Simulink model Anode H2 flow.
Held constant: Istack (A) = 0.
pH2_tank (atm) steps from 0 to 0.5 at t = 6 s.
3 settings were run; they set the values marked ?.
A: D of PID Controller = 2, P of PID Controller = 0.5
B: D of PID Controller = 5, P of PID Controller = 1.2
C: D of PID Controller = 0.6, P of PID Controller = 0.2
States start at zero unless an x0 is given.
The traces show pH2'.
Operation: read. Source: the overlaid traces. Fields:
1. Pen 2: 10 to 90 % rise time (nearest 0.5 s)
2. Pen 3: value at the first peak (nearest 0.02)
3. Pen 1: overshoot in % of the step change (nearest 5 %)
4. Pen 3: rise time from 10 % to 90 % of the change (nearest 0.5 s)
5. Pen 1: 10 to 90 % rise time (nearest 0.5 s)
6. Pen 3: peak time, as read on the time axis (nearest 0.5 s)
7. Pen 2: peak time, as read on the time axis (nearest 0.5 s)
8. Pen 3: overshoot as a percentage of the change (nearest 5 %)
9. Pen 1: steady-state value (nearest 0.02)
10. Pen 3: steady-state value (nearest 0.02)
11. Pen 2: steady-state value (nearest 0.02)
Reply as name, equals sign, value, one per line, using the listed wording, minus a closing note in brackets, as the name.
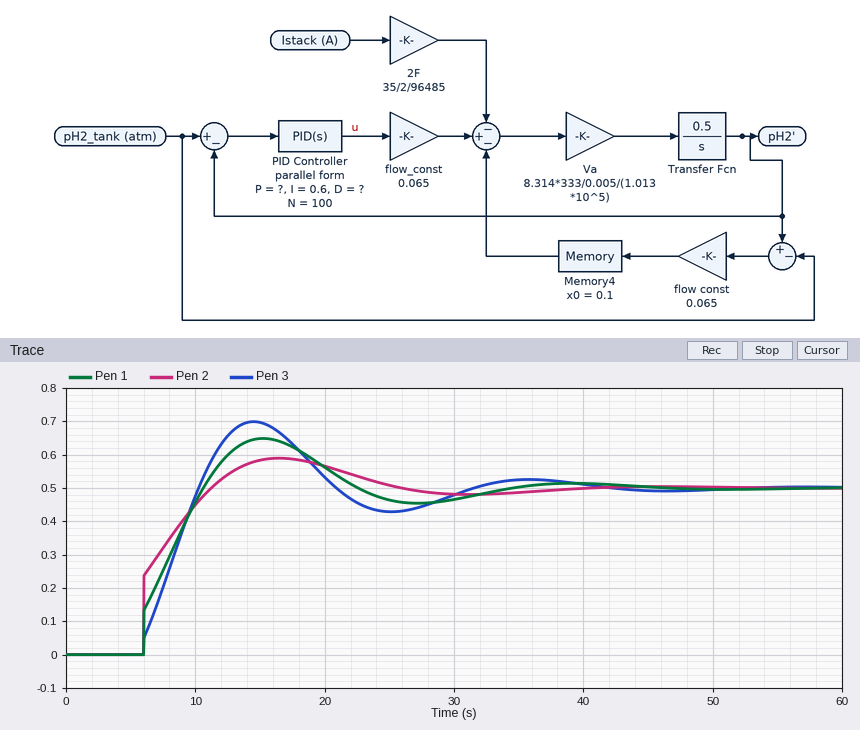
Pen 2: 10 to 90 % rise time = 4.0 s
Pen 3: value at the first peak = 0.70
Pen 1: overshoot in % of the step change = 30 %
Pen 3: rise time from 10 % to 90 % of the change = 3.5 s
Pen 1: 10 to 90 % rise time = 4.0 s
Pen 3: peak time, as read on the time axis = 14.5 s
Pen 2: peak time, as read on the time axis = 16.5 s
Pen 3: overshoot as a percentage of the change = 40 %
Pen 1: steady-state value = 0.50
Pen 3: steady-state value = 0.50
Pen 2: steady-state value = 0.50
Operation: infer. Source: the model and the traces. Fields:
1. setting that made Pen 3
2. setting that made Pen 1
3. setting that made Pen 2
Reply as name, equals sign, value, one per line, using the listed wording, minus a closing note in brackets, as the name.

setting that made Pen 3 = C
setting that made Pen 1 = A
setting that made Pen 2 = B
